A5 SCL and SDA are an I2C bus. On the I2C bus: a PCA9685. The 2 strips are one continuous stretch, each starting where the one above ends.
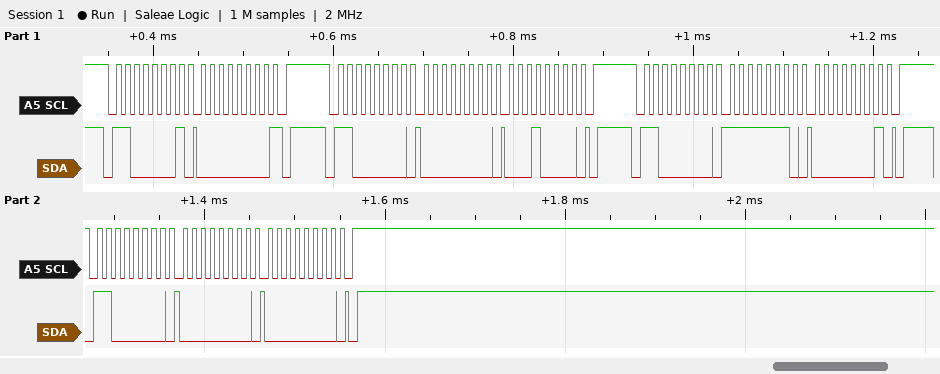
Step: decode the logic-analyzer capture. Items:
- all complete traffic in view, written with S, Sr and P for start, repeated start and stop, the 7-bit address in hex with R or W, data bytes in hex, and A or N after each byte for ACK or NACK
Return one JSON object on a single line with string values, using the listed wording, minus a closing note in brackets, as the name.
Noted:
{"all complete traffic in view, written with S, Sr and P for start, repeated start and stop, the 7-bit address in hex with R or W, data bytes in hex, and A or N after each byte for ACK or NACK": "S 60R A 00 N P S 60W A 00 A 10 A P S 60W A FE A 01 A P S 60W A 00 A 00 A P"}
